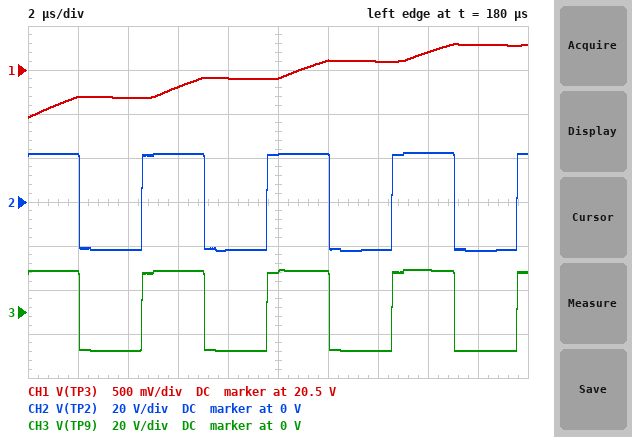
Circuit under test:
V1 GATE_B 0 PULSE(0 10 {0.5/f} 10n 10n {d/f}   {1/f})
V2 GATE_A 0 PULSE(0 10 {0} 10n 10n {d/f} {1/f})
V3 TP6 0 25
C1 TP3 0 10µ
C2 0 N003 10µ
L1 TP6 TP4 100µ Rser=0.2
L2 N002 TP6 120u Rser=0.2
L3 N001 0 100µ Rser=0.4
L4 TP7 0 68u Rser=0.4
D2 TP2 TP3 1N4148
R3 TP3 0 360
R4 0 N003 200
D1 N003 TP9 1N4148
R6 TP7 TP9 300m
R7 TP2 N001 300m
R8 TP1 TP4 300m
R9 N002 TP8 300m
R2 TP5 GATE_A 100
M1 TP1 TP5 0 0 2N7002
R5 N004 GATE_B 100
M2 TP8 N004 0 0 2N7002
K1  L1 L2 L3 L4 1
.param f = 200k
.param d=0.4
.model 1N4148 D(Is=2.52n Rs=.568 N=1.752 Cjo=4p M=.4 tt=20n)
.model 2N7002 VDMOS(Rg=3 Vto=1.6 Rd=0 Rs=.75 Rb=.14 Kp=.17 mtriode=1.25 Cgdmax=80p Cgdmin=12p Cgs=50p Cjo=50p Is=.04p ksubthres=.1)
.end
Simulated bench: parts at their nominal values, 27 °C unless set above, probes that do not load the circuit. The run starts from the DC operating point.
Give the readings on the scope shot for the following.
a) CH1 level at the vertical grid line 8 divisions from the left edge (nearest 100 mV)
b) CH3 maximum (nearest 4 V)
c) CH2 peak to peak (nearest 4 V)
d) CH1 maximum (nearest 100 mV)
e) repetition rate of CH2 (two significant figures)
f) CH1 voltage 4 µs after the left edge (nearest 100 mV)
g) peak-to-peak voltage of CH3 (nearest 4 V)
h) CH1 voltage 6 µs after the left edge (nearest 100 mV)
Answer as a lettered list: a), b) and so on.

a) 20.7 V
b) 20 V
c) 44 V
d) 20.8 V
e) 200 kHz
f) 20.2 V
g) 36 V
h) 20.3 V
